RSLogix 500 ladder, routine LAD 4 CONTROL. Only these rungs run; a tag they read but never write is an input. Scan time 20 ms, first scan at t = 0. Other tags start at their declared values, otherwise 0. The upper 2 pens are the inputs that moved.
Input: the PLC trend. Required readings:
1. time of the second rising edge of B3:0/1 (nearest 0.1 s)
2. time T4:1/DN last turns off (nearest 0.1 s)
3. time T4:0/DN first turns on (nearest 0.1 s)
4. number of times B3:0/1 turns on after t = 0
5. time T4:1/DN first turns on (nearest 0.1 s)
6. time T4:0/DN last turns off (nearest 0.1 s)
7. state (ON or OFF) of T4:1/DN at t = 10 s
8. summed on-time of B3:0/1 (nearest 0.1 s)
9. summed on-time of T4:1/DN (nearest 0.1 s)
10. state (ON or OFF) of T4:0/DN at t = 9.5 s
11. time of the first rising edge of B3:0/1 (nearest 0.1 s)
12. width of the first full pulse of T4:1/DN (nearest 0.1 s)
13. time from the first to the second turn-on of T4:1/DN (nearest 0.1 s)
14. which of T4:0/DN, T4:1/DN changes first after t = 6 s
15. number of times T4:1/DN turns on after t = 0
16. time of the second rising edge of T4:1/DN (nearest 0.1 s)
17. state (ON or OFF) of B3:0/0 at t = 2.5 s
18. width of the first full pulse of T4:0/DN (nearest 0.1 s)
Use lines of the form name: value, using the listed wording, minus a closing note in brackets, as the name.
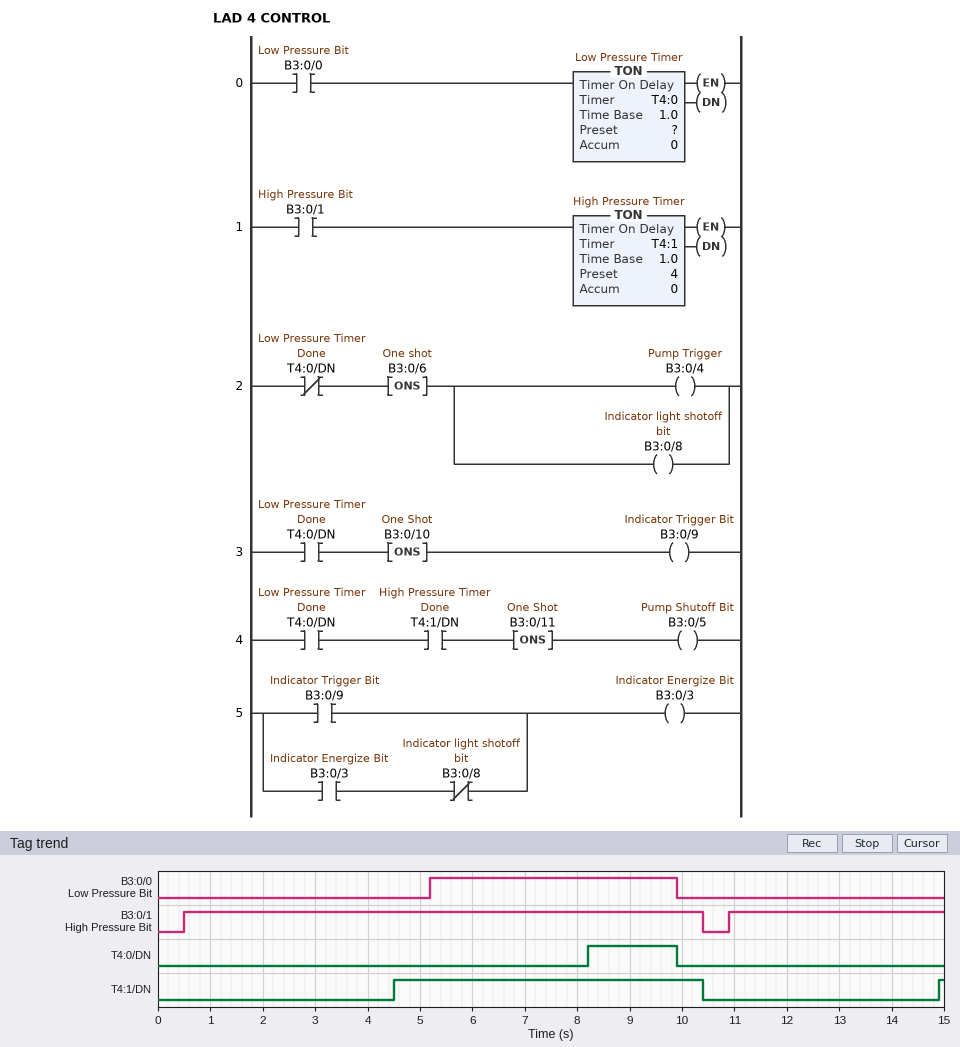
time of the second rising edge of B3:0/1: 10.9 s
time T4:1/DN last turns off: 10.4 s
time T4:0/DN first turns on: 8.2 s
number of times B3:0/1 turns on after t = 0: 2
time T4:1/DN first turns on: 4.5 s
time T4:0/DN last turns off: 9.9 s
state (ON or OFF) of T4:1/DN at t = 10 s: ON
summed on-time of B3:0/1: 14.0 s
summed on-time of T4:1/DN: 6.0 s
state (ON or OFF) of T4:0/DN at t = 9.5 s: ON
time of the first rising edge of B3:0/1: 0.5 s
width of the first full pulse of T4:1/DN: 5.9 s
time from the first to the second turn-on of T4:1/DN: 10.4 s
which of T4:0/DN, T4:1/DN changes first after t = 6 s: T4:0/DN
number of times T4:1/DN turns on after t = 0: 2
time of the second rising edge of T4:1/DN: 14.9 s
state (ON or OFF) of B3:0/0 at t = 2.5 s: OFF
width of the first full pulse of T4:0/DN: 1.7 s
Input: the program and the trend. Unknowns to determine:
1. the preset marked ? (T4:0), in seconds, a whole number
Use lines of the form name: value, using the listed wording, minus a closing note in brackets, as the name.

the preset marked ? (T4:0), in seconds, a whole number: 3 s
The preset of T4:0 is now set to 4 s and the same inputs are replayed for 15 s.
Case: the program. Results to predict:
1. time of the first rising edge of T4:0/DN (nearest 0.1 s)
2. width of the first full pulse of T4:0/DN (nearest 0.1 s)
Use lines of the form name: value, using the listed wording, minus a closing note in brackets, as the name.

time of the first rising edge of T4:0/DN: 9.2 s
width of the first full pulse of T4:0/DN: 0.7 s
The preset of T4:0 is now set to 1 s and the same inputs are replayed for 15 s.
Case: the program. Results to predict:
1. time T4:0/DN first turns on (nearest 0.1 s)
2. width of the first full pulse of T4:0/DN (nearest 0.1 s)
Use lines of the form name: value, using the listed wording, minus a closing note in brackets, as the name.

time T4:0/DN first turns on: 6.2 s
width of the first full pulse of T4:0/DN: 3.7 s
